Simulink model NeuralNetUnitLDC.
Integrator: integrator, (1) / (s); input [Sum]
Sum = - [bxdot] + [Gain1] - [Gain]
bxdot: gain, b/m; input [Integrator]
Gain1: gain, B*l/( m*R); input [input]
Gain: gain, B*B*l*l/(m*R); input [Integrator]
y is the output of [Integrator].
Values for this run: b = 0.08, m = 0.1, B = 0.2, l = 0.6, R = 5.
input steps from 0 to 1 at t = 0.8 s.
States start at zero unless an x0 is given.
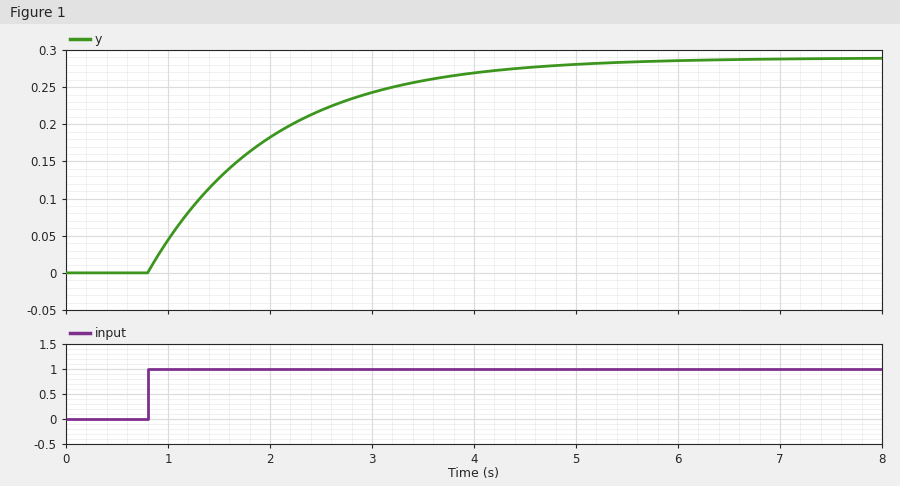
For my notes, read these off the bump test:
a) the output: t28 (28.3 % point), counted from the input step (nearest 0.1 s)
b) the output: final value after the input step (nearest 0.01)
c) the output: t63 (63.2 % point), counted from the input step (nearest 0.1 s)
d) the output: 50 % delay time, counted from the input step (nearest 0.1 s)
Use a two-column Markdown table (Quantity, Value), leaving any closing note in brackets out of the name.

| Quantity | Value |
|---|---|
| the output: t28 (28.3 % point), counted from the input step | 0.4 s |
| the output: final value after the input step | 0.29 |
| the output: t63 (63.2 % point), counted from the input step | 1.2 s |
| the output: 50 % delay time, counted from the input step | 0.8 s |
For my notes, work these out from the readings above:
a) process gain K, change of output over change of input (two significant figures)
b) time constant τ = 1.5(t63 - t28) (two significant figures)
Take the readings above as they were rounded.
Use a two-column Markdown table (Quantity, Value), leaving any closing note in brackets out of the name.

| Quantity | Value |
|---|---|
| process gain K, change of output over change of input | 0.29 |
| time constant τ = 1.5(t63 - t28) | 1.2 s |
